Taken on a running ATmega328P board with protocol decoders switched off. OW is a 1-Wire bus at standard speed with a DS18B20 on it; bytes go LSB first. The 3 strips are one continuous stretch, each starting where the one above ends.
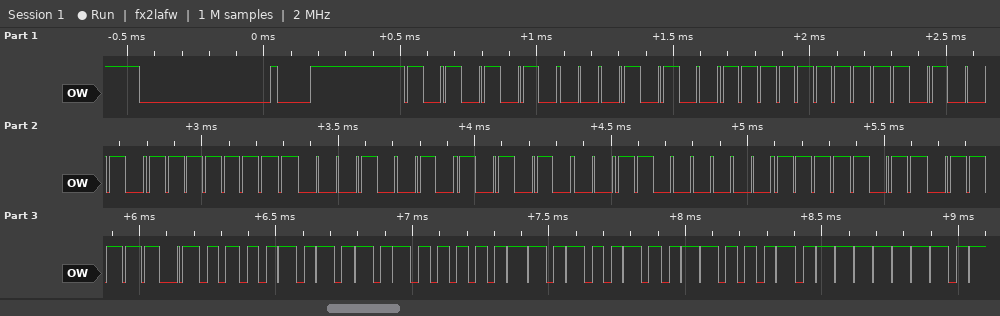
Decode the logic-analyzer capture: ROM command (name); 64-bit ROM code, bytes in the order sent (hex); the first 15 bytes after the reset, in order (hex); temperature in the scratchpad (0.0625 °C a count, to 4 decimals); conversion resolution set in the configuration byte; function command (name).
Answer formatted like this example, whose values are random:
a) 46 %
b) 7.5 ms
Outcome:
a) Match ROM
b) 28 FF 4B FF 48 15 03 DF
c) 55 28 FF 4B FF 48 15 03 DF BE 50 05 4B 46 7F
d) 85.0000 °C
e) 12 bits
f) Read Scratchpad
